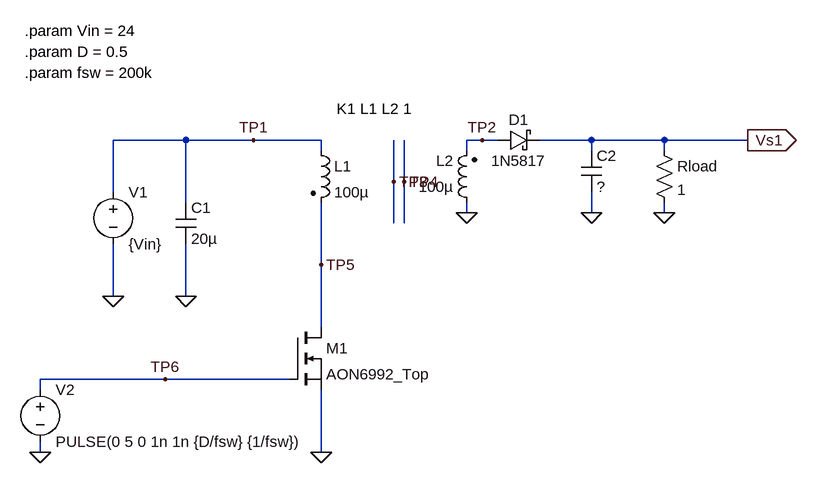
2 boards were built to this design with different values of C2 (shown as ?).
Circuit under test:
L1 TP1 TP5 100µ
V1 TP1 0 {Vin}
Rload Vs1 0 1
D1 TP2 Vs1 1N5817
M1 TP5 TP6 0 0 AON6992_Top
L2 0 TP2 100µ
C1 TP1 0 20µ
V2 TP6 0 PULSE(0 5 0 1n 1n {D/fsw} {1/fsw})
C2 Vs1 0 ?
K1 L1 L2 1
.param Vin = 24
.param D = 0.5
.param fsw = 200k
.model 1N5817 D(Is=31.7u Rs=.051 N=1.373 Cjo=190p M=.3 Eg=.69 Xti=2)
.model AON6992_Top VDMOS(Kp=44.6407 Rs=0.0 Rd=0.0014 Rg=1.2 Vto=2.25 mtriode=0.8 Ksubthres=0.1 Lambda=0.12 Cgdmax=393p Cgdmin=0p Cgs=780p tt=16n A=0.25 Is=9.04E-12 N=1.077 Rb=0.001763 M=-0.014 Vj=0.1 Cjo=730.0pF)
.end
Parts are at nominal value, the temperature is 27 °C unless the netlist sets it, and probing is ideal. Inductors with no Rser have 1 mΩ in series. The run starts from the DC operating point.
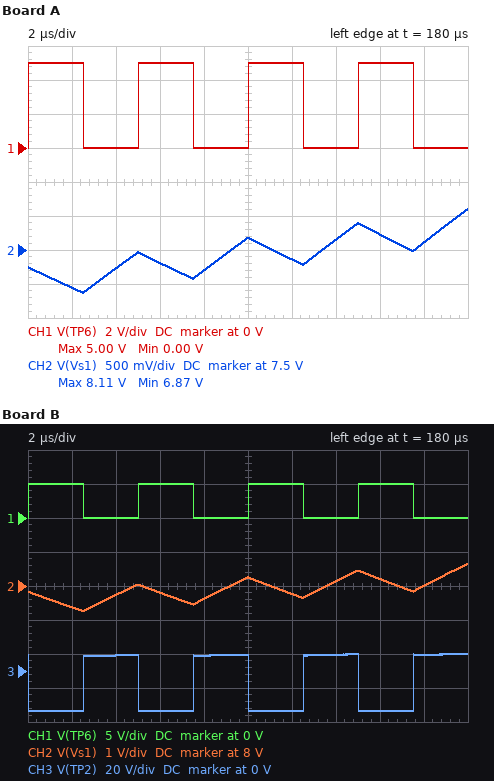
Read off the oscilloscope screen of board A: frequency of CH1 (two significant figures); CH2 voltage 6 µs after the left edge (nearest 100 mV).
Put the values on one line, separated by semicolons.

200 kHz; 7.3 V
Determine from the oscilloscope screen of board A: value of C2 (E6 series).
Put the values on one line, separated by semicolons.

47 µF
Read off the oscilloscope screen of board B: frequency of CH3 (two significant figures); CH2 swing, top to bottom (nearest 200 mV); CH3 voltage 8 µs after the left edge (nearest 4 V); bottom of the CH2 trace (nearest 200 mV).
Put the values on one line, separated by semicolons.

200 kHz; 1.4 V; 8 V; 7.2 V
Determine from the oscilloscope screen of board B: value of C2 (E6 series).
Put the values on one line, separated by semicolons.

33 µF
